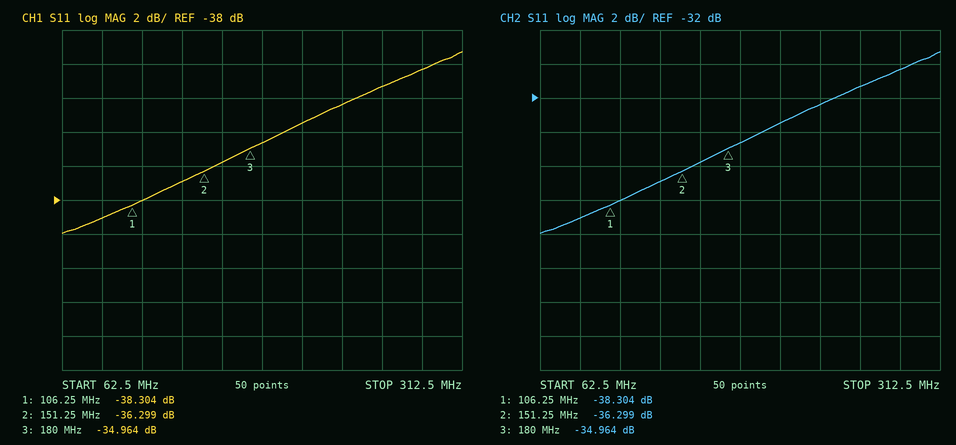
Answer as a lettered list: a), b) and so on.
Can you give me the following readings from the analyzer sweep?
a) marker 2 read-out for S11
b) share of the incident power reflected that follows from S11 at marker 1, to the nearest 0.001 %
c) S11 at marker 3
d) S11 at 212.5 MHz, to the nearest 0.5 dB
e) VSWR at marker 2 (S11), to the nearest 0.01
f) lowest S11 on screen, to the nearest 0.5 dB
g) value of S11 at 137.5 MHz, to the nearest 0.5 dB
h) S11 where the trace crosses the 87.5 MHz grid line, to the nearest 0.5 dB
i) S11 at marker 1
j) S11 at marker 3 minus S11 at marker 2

a) -36.299 dB
b) 0.015 %
c) -34.964 dB
d) -33.5 dB
e) 1.03
f) -40.0 dB
g) -37.0 dB
h) -39.0 dB
i) -38.304 dB
j) 1.335 dB
